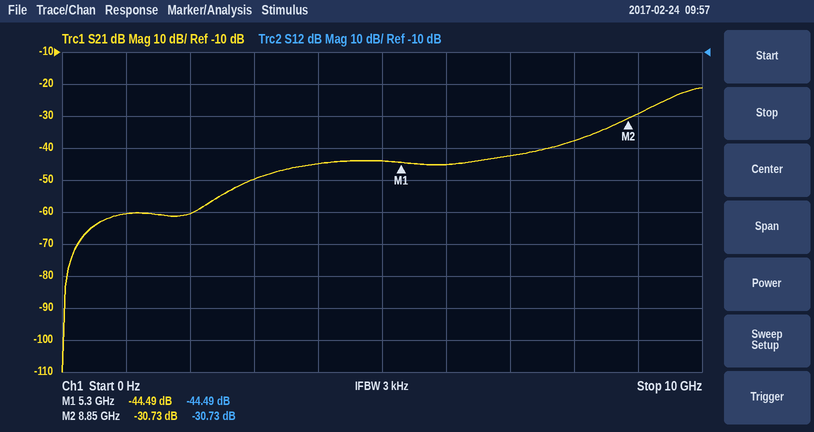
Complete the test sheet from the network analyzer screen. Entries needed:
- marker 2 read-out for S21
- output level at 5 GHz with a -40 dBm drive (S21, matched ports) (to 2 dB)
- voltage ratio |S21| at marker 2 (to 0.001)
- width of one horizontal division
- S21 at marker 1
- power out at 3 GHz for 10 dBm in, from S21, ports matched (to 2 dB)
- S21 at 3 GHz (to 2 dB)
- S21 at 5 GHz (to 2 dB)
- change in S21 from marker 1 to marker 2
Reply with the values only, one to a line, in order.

-30.73 dB
-84 dBm
0.029
1 GHz
-44.49 dB
-40 dBm
-50 dB
-44 dB
13.76 dB
